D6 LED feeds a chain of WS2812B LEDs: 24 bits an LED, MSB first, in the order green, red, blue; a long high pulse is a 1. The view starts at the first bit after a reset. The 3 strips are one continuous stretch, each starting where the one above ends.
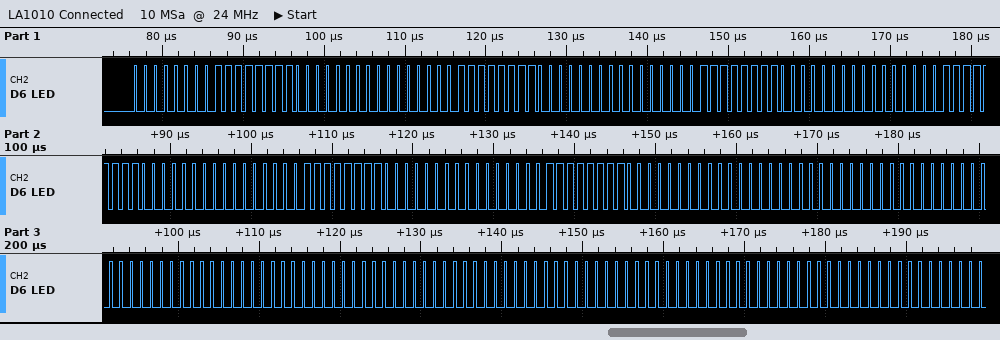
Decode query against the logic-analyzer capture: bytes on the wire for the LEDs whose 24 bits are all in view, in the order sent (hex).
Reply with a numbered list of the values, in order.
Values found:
1. 00 FF 00 00 FF 00 00 FF 00 00 FF 00 00 FF 00 00 FF 00 00 00 00 00 00 00 00 00 00 00 00 00
